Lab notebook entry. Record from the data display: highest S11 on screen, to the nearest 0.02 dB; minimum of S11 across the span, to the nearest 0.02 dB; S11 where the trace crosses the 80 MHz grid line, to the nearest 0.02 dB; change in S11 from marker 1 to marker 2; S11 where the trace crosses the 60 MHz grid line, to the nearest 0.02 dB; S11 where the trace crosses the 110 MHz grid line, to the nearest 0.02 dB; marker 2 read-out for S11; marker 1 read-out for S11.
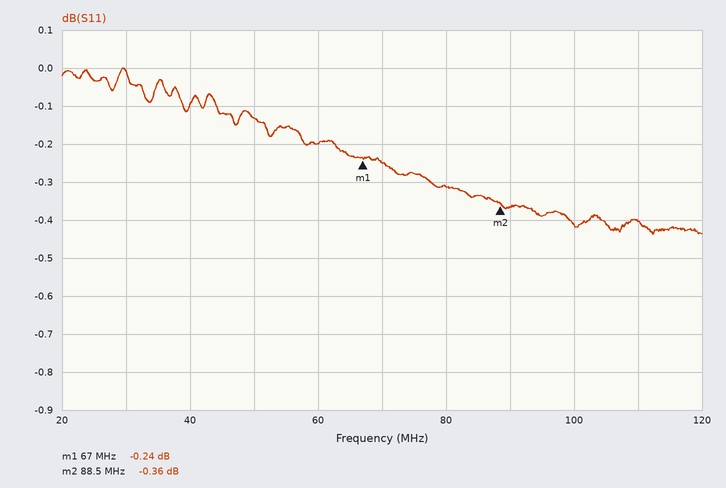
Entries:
0.00 dB
-0.44 dB
-0.32 dB
-0.12 dB
-0.20 dB
-0.40 dB
-0.36 dB
-0.24 dB
